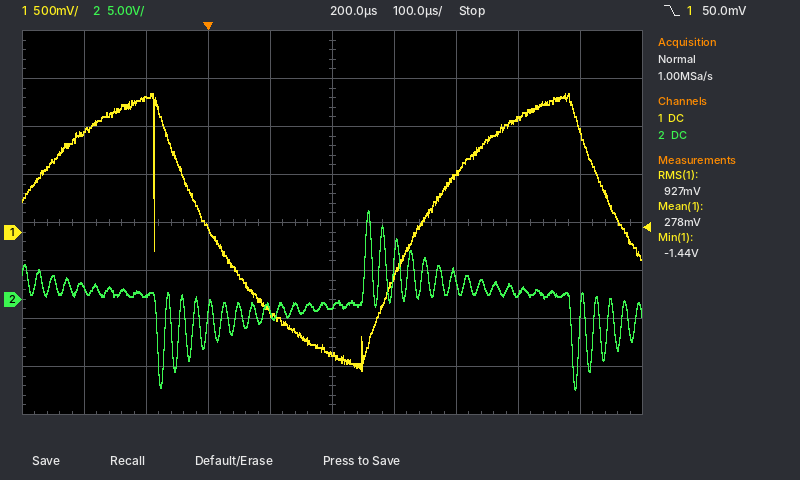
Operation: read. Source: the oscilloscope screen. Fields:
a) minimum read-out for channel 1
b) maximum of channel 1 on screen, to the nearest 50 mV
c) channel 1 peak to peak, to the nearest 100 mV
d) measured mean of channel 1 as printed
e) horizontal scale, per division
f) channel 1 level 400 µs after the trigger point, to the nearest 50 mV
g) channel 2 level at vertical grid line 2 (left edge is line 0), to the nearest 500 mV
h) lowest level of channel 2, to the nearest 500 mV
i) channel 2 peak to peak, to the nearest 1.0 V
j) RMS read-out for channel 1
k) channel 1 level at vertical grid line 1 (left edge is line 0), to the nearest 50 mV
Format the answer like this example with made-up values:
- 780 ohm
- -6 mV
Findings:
- -1.44 V
- 1.45 V
- 2.90 V
- 278 mV
- 100 µs
- 600 mV
- 500 mV
- -9.5 V
- 19.0 V
- 927 mV
- 1.05 V
